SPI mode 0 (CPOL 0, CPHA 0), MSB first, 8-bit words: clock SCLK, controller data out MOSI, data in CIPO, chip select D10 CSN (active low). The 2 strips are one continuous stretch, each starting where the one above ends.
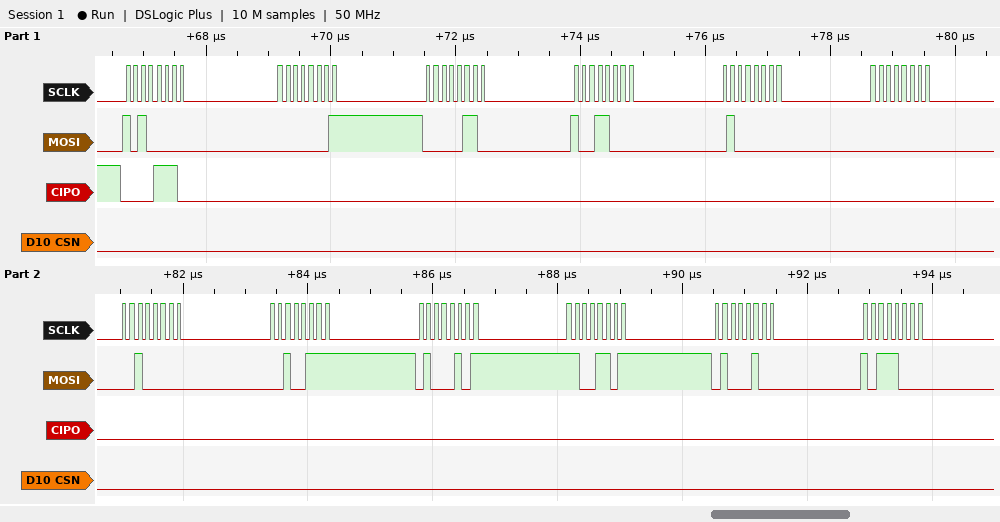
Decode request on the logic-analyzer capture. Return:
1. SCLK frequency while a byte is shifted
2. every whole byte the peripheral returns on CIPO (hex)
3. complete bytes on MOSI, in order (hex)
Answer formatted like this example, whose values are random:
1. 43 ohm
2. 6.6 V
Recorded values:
1. 8 MHz
2. 0E 00 00 00 00 00 00 00 00 00 00 00
3. A0 01 06 98 40 00 20 27 45 CD 44 B8
